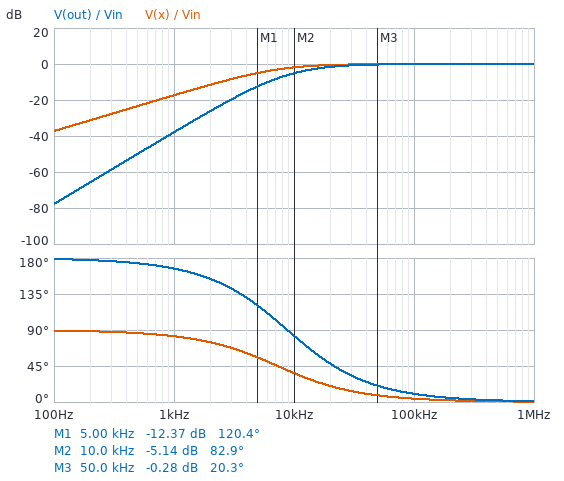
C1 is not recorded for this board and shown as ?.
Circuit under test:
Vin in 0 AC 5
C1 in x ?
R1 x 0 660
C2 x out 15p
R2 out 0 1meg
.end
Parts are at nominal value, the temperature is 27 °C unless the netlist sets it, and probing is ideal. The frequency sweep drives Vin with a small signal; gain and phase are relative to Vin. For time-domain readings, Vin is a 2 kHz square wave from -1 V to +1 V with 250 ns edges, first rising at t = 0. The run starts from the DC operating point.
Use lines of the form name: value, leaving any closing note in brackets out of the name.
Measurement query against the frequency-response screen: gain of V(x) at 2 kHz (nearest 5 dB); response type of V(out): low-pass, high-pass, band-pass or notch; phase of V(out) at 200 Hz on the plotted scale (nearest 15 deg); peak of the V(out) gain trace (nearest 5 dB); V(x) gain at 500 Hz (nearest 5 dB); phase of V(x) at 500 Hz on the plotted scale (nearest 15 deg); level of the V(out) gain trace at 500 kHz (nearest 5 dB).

gain of V(x) at 2 kHz: -10 dB
response type of V(out): low-pass, high-pass, band-pass or notch: high-pass
phase of V(out) at 200 Hz on the plotted scale: 180 deg
peak of the V(out) gain trace: 0 dB
V(x) gain at 500 Hz: -25 dB
phase of V(x) at 500 Hz on the plotted scale: 90 deg
level of the V(out) gain trace at 500 kHz: 0 dB
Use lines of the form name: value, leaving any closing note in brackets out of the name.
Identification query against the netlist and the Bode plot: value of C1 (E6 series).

value of C1: 33 nF
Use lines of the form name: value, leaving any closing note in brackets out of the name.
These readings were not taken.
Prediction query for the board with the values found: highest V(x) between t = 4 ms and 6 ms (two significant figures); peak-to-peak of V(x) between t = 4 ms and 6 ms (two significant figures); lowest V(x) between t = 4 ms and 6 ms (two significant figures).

highest V(x) between t = 4 ms and 6 ms: 2.0 V
peak-to-peak of V(x) between t = 4 ms and 6 ms: 4.0 V
lowest V(x) between t = 4 ms and 6 ms: -2.0 V
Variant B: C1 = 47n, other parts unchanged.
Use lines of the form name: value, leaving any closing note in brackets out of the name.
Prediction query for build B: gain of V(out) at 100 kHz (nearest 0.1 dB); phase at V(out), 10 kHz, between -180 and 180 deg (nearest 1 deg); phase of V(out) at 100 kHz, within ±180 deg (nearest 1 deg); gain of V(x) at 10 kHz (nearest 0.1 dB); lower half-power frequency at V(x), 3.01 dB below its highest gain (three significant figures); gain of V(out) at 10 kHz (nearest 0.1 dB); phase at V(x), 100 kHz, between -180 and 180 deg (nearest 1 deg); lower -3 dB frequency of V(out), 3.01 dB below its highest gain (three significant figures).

gain of V(out) at 100 kHz: -0.1 dB
phase at V(out), 10 kHz, between -180 and 180 deg: 74 deg
phase of V(out) at 100 kHz, within ±180 deg: 9 deg
gain of V(x) at 10 kHz: -1.0 dB
lower half-power frequency at V(x), 3.01 dB below its highest gain: 5.13 kHz
gain of V(out) at 10 kHz: -4.3 dB
phase at V(x), 100 kHz, between -180 and 180 deg: 3 deg
lower -3 dB frequency of V(out), 3.01 dB below its highest gain: 12.6 kHz
